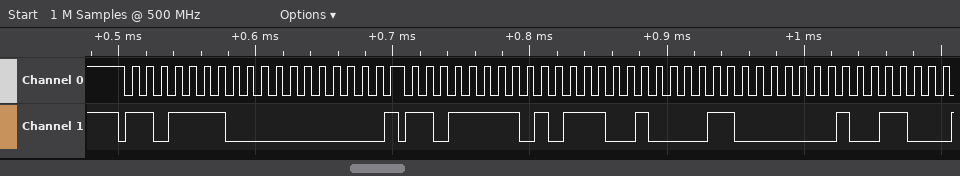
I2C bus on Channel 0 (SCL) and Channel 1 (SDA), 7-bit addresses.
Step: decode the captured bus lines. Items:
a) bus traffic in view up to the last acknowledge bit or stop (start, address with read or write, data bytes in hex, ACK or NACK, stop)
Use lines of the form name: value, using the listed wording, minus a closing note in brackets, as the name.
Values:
bus traffic in view up to the last acknowledge bit or stop: start, address 6F write ACK, 00 ACK, repeated start, address 6F read ACK, B9 ACK, 18 ACK, 13 ACK
